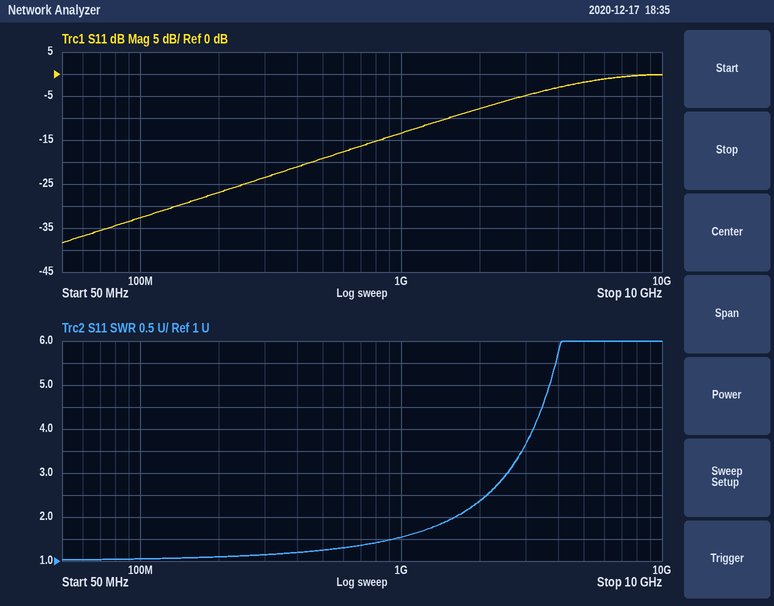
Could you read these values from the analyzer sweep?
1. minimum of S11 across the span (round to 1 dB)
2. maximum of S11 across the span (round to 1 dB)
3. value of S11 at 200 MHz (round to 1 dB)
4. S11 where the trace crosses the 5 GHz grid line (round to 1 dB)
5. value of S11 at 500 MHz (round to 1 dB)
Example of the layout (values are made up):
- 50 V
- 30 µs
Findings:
- -38 dB
- 0 dB
- -27 dB
- -2 dB
- -19 dB
